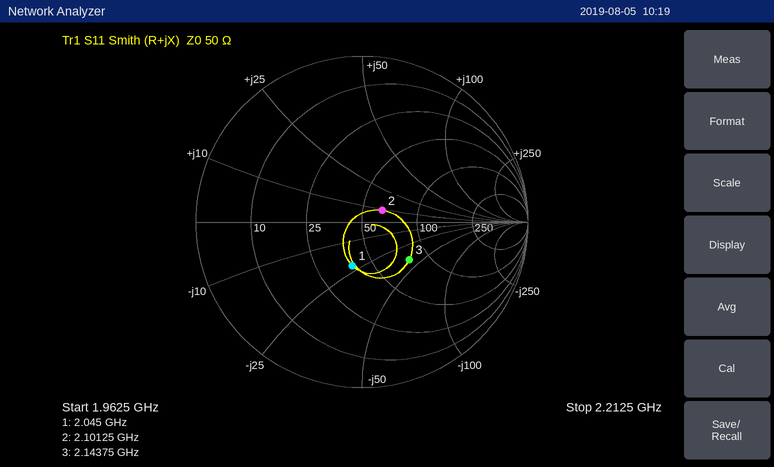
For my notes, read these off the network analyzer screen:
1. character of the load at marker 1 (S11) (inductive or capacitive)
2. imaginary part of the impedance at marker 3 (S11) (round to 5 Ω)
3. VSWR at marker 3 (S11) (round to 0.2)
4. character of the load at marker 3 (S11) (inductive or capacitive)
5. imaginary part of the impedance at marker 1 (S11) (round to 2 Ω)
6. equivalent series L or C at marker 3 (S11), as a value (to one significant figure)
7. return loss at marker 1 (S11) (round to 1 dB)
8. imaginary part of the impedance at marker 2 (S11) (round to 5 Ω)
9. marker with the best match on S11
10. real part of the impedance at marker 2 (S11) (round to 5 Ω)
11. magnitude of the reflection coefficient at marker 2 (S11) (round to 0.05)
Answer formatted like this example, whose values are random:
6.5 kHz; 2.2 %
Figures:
capacitive; -40 Ω; 2.2; capacitive; -22 Ω; 2 pF; 11 dB; +10 Ω; marker 2; 65 Ω; 0.15
